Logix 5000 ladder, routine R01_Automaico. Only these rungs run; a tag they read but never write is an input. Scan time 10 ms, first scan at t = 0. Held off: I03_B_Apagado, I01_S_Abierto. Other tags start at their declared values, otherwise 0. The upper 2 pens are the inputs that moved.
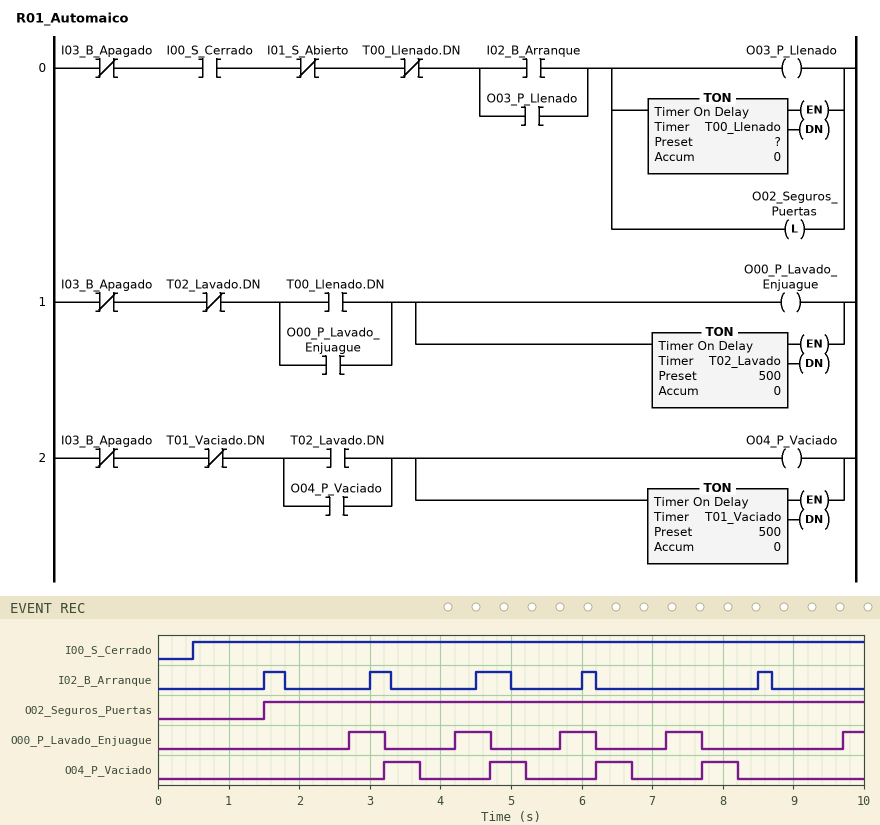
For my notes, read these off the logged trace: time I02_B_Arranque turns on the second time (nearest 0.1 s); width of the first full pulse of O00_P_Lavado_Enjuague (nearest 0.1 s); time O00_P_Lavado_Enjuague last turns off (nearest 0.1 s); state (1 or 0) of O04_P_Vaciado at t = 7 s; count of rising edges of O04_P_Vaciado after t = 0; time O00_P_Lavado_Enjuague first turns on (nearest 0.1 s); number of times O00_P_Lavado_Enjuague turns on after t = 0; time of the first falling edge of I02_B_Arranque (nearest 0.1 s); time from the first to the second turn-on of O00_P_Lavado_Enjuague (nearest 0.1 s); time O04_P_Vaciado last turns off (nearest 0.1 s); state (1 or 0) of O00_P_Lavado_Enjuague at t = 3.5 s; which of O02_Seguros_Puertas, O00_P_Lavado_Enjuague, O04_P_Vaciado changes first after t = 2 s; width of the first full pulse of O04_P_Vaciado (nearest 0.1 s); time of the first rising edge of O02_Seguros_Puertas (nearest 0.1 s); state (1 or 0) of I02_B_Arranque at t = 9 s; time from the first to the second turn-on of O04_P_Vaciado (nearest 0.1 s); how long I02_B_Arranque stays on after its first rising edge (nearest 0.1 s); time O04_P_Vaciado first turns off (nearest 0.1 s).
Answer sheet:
3.0 s
0.5 s
7.7 s
0
4
2.7 s
5
1.8 s
1.5 s
8.2 s
0
O00_P_Lavado_Enjuague
0.5 s
1.5 s
0
1.5 s
0.3 s
3.7 s
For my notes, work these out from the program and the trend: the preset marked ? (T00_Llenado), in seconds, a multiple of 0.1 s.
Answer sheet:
1.2 s
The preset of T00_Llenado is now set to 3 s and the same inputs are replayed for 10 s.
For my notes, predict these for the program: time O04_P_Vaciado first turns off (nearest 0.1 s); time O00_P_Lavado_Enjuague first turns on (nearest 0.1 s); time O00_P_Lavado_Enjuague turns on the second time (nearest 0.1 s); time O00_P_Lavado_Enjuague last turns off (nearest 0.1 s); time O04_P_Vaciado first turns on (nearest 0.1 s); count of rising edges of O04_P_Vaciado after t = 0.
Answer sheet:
5.5 s
4.5 s
7.5 s
8.0 s
5.0 s
2
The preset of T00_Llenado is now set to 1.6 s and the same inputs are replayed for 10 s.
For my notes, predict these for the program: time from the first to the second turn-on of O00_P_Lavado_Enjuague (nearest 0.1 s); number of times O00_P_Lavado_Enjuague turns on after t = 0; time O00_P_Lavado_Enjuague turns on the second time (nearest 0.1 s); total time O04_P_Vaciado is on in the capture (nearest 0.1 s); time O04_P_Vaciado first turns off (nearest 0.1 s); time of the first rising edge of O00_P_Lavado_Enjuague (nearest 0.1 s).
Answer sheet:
1.6 s
3
4.7 s
1.5 s
4.1 s
3.1 s
